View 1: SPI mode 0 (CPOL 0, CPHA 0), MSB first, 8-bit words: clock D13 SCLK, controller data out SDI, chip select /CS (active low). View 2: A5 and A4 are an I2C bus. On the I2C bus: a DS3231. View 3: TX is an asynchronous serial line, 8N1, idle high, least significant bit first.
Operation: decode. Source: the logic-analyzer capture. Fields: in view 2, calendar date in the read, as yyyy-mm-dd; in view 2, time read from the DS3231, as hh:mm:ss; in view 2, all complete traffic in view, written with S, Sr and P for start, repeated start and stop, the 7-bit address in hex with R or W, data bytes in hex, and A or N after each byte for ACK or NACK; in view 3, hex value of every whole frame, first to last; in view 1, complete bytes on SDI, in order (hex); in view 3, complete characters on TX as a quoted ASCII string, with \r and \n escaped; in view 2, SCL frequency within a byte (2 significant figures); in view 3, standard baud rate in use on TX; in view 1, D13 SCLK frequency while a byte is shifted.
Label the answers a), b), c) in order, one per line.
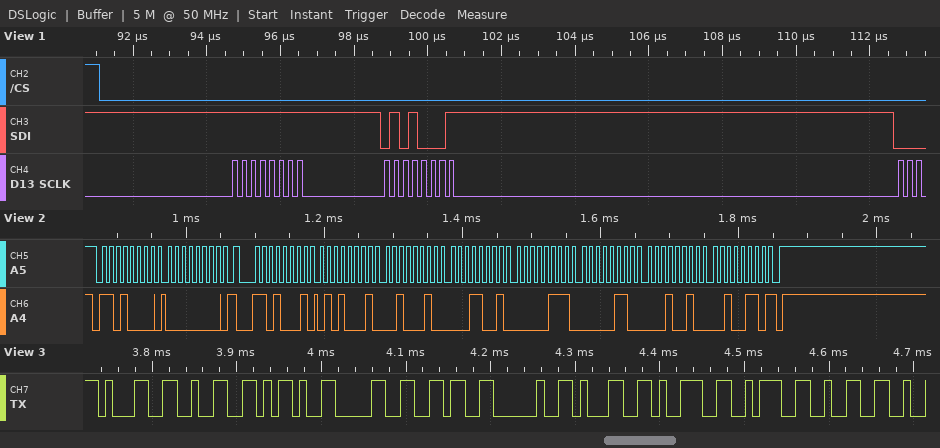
a) 2026-12-06
b) 19:22:51
c) S 68W A 00 A Sr 68R A 51 A 22 A 19 A 07 A 06 A 12 A 26 N P
d) 31 32 2D 30 36 20 31 39 3A 32
e) FF 51
f) "12-06 19:2"
g) 100 kHz
h) 115200 baud
i) 4 MHz
